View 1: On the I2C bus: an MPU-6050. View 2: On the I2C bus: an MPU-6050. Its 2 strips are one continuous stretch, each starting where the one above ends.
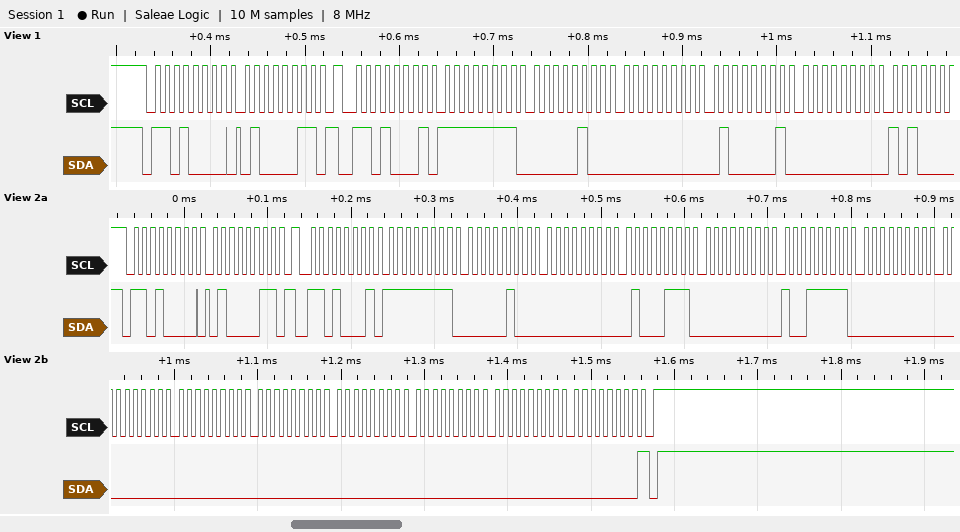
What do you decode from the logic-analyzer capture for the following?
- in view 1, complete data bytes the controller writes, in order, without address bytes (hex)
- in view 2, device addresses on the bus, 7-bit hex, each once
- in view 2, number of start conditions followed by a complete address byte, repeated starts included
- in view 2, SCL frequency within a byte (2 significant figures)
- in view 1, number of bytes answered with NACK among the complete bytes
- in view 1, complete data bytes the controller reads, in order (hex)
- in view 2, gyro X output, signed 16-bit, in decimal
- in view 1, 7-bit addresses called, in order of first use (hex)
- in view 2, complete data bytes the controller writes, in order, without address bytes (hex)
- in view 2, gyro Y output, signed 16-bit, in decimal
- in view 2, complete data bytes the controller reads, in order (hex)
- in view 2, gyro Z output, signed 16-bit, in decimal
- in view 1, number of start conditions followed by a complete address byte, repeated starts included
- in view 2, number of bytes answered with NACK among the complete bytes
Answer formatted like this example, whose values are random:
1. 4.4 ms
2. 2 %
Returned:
1. 43
2. 0x68
3. 2
4. 100 kHz
5. 0
6. FF 04 00 41 00
7. -252
8. 0x68
9. 43
10. 71
11. FF 04 00 47 00 9F 00 00 00 00 00 00 00 00
12. 159
13. 2
14. 1
